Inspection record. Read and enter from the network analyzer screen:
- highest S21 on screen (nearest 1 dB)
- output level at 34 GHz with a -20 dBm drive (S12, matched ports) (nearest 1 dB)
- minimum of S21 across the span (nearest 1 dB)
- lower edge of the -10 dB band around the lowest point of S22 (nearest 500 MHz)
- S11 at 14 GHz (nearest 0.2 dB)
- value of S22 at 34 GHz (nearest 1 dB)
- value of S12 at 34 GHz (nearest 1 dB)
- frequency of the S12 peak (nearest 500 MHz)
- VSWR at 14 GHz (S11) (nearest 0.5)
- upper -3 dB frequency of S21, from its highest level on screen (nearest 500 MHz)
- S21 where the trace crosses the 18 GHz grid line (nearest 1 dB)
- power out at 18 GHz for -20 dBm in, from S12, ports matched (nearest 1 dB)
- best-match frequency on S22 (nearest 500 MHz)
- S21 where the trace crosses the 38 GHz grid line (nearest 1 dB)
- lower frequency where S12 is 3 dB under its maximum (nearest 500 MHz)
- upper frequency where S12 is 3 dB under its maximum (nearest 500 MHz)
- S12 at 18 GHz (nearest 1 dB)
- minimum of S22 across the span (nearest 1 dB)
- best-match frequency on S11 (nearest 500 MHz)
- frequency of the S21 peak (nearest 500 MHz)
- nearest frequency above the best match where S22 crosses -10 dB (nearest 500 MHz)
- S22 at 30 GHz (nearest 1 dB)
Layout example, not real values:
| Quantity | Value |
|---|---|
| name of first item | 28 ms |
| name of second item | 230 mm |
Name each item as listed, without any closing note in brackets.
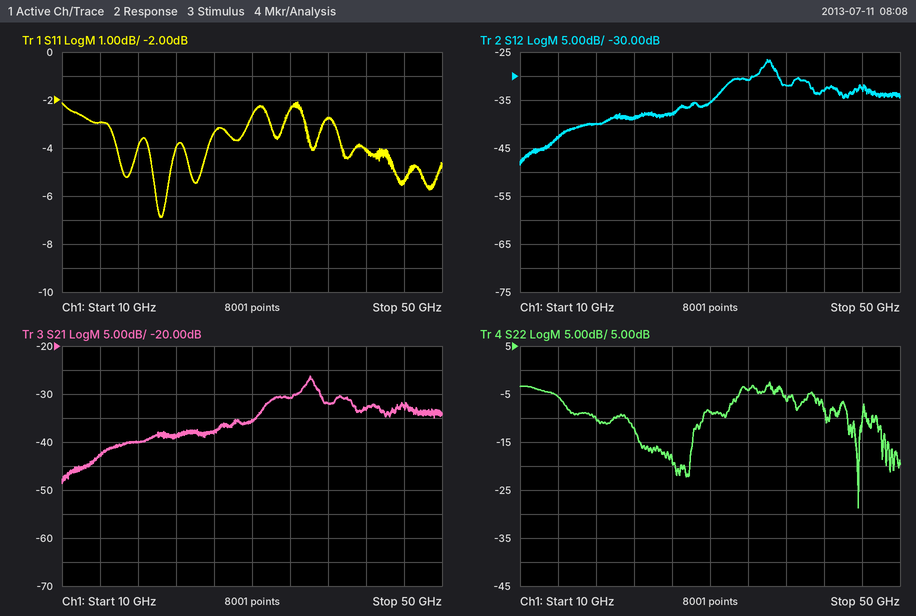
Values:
| Quantity | Value |
|---|---|
| highest S21 on screen | -26 dB |
| output level at 34 GHz with a -20 dBm drive (S12, matched ports) | -51 dBm |
| minimum of S21 across the span | -49 dB |
| lower edge of the -10 dB band around the lowest point of S22 | 44.5 GHz |
| S11 at 14 GHz | -3.0 dB |
| value of S22 at 34 GHz | -4 dB |
| value of S12 at 34 GHz | -31 dB |
| frequency of the S12 peak | 36.0 GHz |
| VSWR at 14 GHz (S11) | 6.0 |
| upper -3 dB frequency of S21, from its highest level on screen | 37.0 GHz |
| S21 where the trace crosses the 18 GHz grid line | -40 dB |
| power out at 18 GHz for -20 dBm in, from S12, ports matched | -60 dBm |
| best-match frequency on S22 | 45.5 GHz |
| S21 where the trace crosses the 38 GHz grid line | -32 dB |
| lower frequency where S12 is 3 dB under its maximum | 35.0 GHz |
| upper frequency where S12 is 3 dB under its maximum | 37.0 GHz |
| S12 at 18 GHz | -40 dB |
| minimum of S22 across the span | -29 dB |
| best-match frequency on S11 | 20.5 GHz |
| frequency of the S21 peak | 36.0 GHz |
| nearest frequency above the best match where S22 crosses -10 dB | 46.0 GHz |
| S22 at 30 GHz | -9 dB |
